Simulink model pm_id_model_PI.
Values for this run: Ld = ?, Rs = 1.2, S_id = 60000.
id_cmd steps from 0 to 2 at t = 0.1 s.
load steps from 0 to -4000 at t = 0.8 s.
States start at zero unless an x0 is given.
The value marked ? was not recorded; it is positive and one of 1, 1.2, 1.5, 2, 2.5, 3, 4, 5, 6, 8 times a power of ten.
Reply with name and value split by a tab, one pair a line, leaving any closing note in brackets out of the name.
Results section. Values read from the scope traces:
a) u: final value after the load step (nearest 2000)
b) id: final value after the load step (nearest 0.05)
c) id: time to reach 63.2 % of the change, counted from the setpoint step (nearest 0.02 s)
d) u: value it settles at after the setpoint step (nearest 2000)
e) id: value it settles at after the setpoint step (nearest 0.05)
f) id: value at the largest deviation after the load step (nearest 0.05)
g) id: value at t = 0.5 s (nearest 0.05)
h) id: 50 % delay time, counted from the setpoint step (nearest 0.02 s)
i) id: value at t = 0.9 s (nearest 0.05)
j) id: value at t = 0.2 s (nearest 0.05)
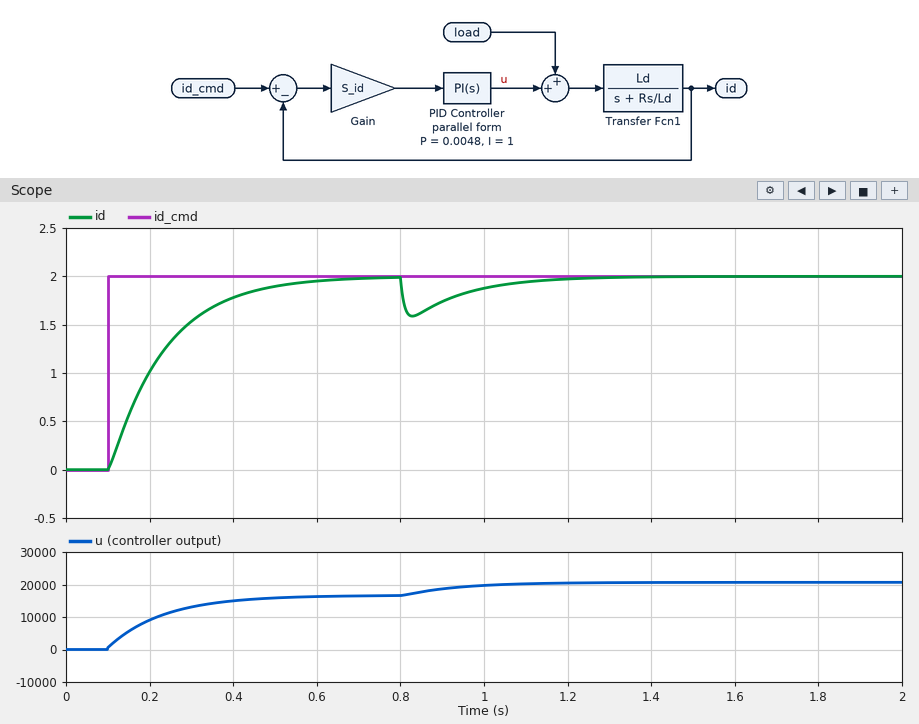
u: final value after the load step	20000
id: final value after the load step	2.00
id: time to reach 63.2 % of the change, counted from the setpoint step	0.14 s
u: value it settles at after the setpoint step	16000
id: value it settles at after the setpoint step	2.00
id: value at the largest deviation after the load step	1.60
id: value at t = 0.5 s	1.90
id: 50 % delay time, counted from the setpoint step	0.10 s
id: value at t = 0.9 s	1.75
id: value at t = 0.2 s	1.00
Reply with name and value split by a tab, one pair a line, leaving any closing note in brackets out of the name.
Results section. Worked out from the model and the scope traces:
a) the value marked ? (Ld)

the value marked ?	0.012
